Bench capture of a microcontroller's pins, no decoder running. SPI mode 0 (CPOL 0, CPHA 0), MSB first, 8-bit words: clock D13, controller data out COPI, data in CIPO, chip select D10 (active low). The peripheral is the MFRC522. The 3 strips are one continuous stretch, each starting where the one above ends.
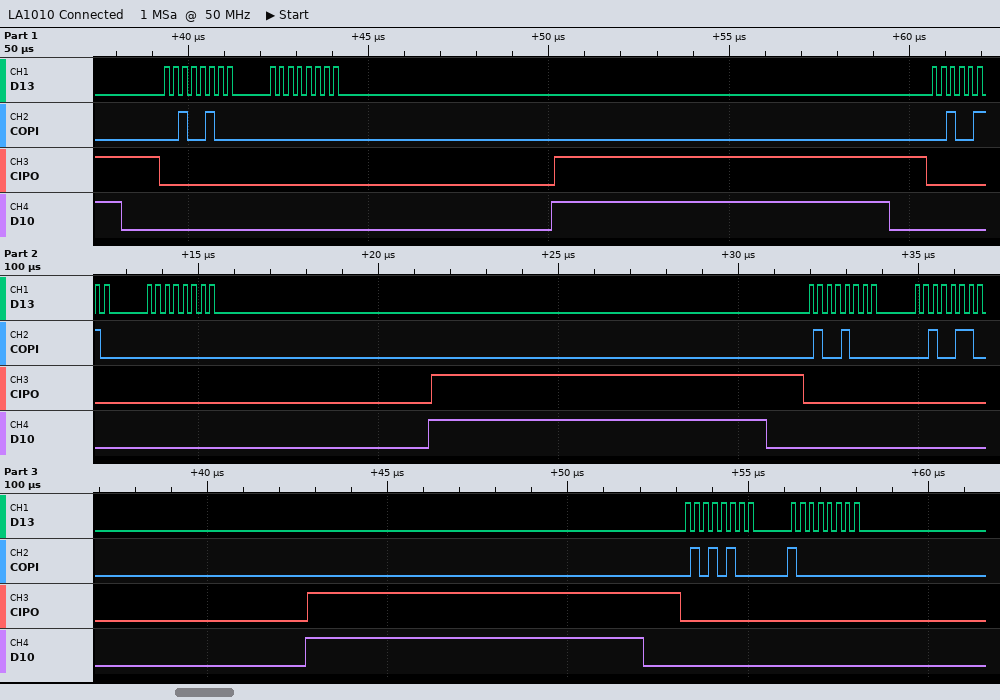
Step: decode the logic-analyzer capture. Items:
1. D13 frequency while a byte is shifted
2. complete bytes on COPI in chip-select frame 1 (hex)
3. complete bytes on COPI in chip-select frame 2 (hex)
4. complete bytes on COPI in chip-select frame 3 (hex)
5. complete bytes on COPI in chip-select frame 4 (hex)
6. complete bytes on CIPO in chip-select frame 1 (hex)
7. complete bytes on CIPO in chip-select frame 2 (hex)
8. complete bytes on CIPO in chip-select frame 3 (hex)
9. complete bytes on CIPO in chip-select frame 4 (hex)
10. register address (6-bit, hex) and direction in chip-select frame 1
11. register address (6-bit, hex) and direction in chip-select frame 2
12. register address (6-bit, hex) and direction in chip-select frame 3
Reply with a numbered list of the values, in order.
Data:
1. 4 MHz
2. 0x24 0x00
3. 0x26 0x00
4. 0x48 0x26
5. 0x54 0x80
6. 0x00 0x00
7. 0x00 0x00
8. 0x00 0x00
9. 0x00 0x00
10. 0x12 write
11. 0x13 write
12. 0x24 write
